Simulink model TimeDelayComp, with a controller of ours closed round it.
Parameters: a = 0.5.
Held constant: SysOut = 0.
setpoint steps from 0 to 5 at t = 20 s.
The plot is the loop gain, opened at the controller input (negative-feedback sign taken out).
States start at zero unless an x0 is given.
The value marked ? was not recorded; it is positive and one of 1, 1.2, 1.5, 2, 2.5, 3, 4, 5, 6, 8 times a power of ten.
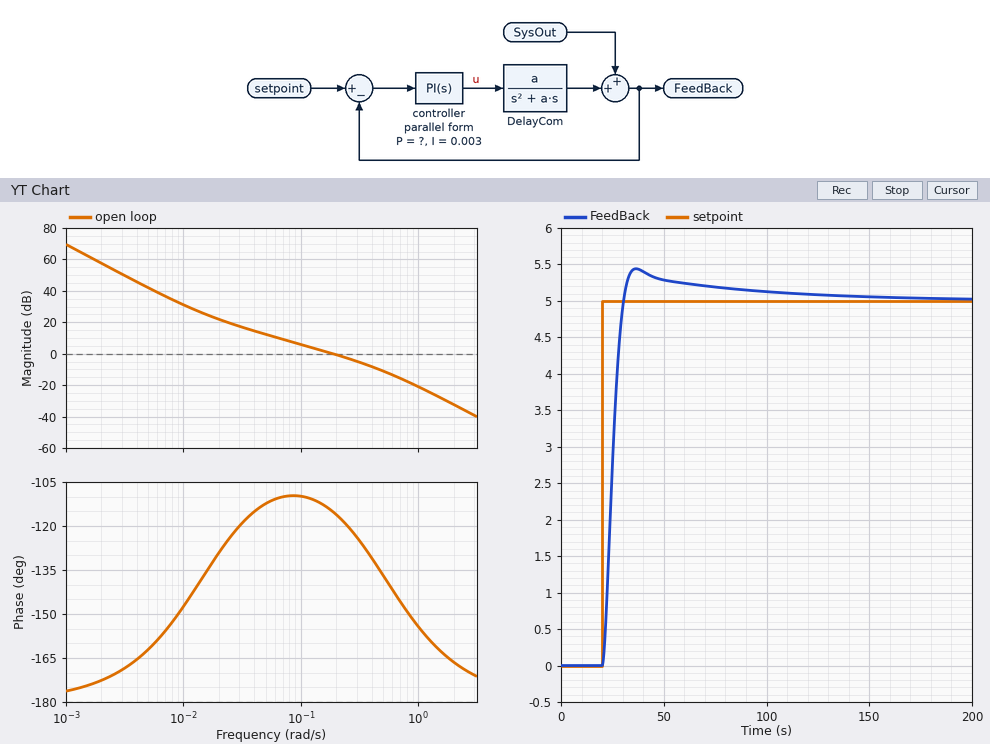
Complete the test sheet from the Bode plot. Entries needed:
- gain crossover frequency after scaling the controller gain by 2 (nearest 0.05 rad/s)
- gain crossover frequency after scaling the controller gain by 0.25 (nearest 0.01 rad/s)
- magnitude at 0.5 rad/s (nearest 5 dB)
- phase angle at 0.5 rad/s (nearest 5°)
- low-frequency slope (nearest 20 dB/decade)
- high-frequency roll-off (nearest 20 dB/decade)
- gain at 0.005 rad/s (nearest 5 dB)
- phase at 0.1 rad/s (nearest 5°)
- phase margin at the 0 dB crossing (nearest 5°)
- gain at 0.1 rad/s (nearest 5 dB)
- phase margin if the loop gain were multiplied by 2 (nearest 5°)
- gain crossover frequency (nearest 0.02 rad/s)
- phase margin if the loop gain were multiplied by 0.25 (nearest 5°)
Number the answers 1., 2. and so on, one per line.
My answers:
1. 0.35 rad/s
2. 0.05 rad/s
3. -10 dB
4. -135°
5. -40 dB/decade
6. -40 dB/decade
7. 40 dB
8. -110°
9. 65°
10. 5 dB
11. 55°
12. 0.18 rad/s
13. 70°
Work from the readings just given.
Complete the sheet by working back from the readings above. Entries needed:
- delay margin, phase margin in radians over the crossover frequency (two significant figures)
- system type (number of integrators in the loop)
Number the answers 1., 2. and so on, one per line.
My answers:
1. 6.3 s
2. 2
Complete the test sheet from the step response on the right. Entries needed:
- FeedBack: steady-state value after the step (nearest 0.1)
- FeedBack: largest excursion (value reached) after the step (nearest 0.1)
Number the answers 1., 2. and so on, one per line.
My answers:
1. 5.0
2. 5.4
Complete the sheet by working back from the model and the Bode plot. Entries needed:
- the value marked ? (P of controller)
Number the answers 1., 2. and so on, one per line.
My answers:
1. 0.2
